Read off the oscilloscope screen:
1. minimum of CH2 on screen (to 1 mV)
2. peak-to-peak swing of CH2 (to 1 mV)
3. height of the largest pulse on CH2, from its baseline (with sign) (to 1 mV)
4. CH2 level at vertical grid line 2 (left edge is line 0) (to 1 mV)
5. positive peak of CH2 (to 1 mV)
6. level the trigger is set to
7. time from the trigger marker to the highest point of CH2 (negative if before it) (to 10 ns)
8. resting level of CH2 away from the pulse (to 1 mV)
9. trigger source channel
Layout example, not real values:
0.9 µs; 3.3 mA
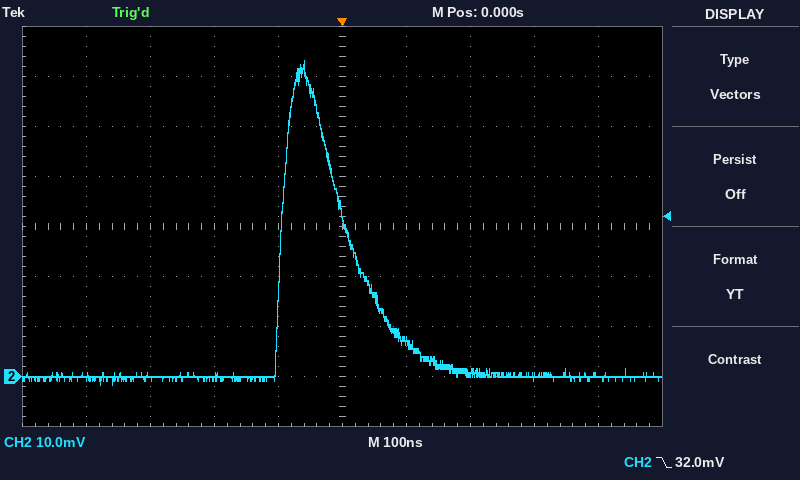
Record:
-2 mV; 65 mV; +63 mV; 0 mV; 63 mV; 32.0 mV; -60 ns; 0 mV; CH2
